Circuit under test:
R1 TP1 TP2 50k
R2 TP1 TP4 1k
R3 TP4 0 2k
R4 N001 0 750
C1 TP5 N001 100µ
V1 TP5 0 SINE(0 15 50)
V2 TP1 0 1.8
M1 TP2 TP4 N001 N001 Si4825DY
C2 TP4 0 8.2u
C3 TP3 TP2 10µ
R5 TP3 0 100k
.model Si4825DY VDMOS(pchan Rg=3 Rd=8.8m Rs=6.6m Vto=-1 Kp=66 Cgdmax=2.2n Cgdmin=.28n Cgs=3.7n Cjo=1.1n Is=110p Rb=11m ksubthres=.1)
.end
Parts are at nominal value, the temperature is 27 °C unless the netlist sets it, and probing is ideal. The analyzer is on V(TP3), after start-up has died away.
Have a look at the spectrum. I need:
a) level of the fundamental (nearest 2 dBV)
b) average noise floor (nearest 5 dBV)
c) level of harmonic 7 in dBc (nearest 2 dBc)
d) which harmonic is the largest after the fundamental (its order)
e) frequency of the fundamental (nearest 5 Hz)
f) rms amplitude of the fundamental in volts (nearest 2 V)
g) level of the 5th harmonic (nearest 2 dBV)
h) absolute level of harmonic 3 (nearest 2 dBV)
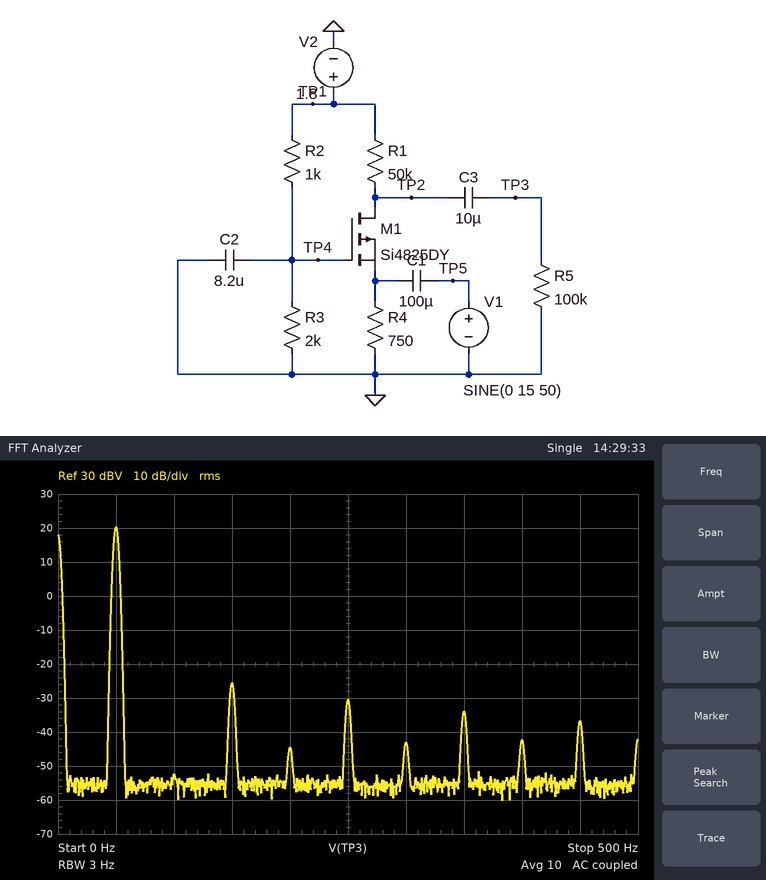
20 dBV
-55 dBV
-54 dBc
3
50 Hz
10 V
-30 dBV
-26 dBV
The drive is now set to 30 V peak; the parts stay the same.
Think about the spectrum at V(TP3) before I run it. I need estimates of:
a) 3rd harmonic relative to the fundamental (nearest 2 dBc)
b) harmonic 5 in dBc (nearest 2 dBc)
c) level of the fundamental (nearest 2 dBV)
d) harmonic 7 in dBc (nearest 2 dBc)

-52 dBc
-56 dBc
26 dBV
-60 dBc
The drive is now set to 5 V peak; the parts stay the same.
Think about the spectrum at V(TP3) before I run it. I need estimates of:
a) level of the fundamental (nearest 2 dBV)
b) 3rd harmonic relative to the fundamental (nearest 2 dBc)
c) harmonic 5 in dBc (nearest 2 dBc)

10 dBV
-38 dBc
-44 dBc
